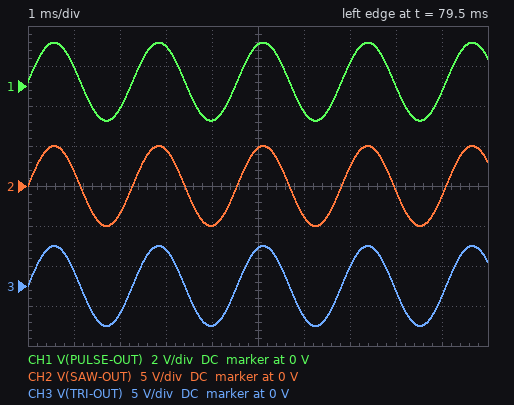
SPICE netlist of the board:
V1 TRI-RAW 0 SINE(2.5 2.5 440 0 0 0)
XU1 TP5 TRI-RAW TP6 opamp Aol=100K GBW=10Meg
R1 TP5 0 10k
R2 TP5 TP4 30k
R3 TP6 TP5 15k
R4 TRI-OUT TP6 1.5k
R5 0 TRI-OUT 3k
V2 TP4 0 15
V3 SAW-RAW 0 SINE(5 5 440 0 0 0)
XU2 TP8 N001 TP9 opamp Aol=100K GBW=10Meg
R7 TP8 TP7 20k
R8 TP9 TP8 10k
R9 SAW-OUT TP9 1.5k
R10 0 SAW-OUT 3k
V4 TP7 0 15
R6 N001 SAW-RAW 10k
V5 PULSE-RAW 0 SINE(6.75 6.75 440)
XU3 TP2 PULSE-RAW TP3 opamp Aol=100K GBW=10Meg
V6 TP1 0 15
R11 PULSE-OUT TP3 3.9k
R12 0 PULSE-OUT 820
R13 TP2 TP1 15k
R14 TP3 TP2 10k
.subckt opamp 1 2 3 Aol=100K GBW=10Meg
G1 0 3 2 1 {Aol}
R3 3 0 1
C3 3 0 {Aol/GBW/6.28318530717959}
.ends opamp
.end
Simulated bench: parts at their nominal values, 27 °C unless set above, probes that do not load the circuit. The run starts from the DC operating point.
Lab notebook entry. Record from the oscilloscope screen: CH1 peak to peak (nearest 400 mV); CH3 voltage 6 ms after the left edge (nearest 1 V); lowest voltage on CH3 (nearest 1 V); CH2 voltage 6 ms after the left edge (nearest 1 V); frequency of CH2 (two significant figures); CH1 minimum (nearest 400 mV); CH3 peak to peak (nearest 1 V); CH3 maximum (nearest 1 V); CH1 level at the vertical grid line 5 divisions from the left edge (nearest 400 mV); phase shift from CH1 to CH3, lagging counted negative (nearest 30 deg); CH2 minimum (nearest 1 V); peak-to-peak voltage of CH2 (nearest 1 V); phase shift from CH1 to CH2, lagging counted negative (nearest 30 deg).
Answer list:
4.0 V
-4 V
-5 V
-4 V
440 Hz
-1.6 V
10 V
5 V
2.0 V
0 deg
-5 V
10 V
0 deg
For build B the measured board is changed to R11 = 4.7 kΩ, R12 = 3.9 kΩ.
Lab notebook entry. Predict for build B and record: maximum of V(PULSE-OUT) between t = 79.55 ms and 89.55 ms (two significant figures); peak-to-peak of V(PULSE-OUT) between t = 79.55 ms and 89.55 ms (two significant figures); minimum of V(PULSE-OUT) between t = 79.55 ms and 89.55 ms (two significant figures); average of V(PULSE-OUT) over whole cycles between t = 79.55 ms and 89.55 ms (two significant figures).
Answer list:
5.7 V
10 V
-4.5 V
570 mV
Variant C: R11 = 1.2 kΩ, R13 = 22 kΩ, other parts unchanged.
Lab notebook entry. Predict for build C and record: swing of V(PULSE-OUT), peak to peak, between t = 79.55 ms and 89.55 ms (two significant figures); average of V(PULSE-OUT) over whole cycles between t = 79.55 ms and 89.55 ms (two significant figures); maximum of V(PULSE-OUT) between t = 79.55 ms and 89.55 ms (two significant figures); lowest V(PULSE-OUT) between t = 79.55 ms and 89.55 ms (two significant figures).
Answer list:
8.0 V
1.2 V
5.2 V
-2.8 V
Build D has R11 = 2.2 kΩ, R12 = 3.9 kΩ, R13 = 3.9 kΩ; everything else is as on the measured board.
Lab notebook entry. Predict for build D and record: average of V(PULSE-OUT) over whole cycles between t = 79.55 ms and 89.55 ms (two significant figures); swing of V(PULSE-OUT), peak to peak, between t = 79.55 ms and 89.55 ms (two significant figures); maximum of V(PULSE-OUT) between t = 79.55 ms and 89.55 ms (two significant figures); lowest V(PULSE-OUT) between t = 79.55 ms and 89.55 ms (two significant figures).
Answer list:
-9.2 V
31 V
6.2 V
-25 V
